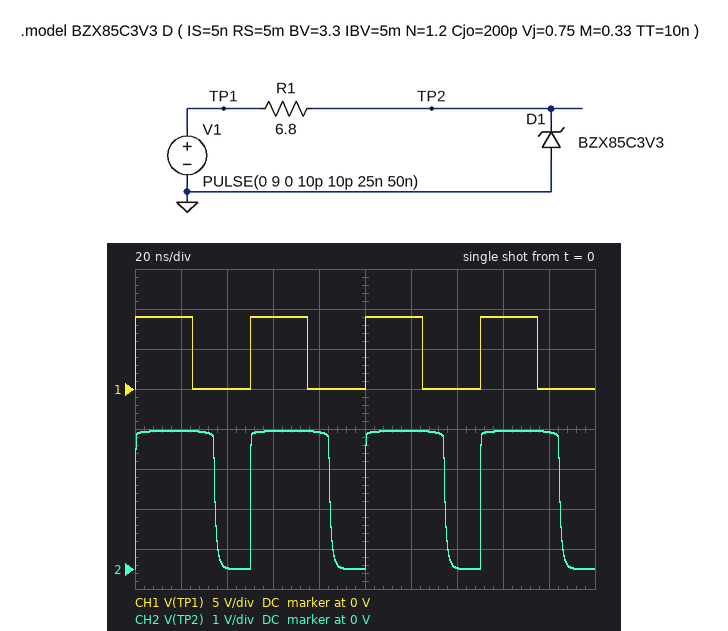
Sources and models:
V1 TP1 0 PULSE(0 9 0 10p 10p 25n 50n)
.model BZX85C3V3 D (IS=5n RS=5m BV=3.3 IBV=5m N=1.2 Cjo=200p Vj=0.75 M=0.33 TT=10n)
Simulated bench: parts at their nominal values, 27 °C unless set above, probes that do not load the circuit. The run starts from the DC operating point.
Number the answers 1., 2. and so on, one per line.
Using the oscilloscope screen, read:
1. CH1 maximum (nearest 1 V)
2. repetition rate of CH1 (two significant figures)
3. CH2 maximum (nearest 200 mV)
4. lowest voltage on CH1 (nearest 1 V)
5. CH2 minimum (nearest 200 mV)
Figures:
1. 9 V
2. 20 MHz
3. 3.4 V
4. 0 V
5. 0 V
